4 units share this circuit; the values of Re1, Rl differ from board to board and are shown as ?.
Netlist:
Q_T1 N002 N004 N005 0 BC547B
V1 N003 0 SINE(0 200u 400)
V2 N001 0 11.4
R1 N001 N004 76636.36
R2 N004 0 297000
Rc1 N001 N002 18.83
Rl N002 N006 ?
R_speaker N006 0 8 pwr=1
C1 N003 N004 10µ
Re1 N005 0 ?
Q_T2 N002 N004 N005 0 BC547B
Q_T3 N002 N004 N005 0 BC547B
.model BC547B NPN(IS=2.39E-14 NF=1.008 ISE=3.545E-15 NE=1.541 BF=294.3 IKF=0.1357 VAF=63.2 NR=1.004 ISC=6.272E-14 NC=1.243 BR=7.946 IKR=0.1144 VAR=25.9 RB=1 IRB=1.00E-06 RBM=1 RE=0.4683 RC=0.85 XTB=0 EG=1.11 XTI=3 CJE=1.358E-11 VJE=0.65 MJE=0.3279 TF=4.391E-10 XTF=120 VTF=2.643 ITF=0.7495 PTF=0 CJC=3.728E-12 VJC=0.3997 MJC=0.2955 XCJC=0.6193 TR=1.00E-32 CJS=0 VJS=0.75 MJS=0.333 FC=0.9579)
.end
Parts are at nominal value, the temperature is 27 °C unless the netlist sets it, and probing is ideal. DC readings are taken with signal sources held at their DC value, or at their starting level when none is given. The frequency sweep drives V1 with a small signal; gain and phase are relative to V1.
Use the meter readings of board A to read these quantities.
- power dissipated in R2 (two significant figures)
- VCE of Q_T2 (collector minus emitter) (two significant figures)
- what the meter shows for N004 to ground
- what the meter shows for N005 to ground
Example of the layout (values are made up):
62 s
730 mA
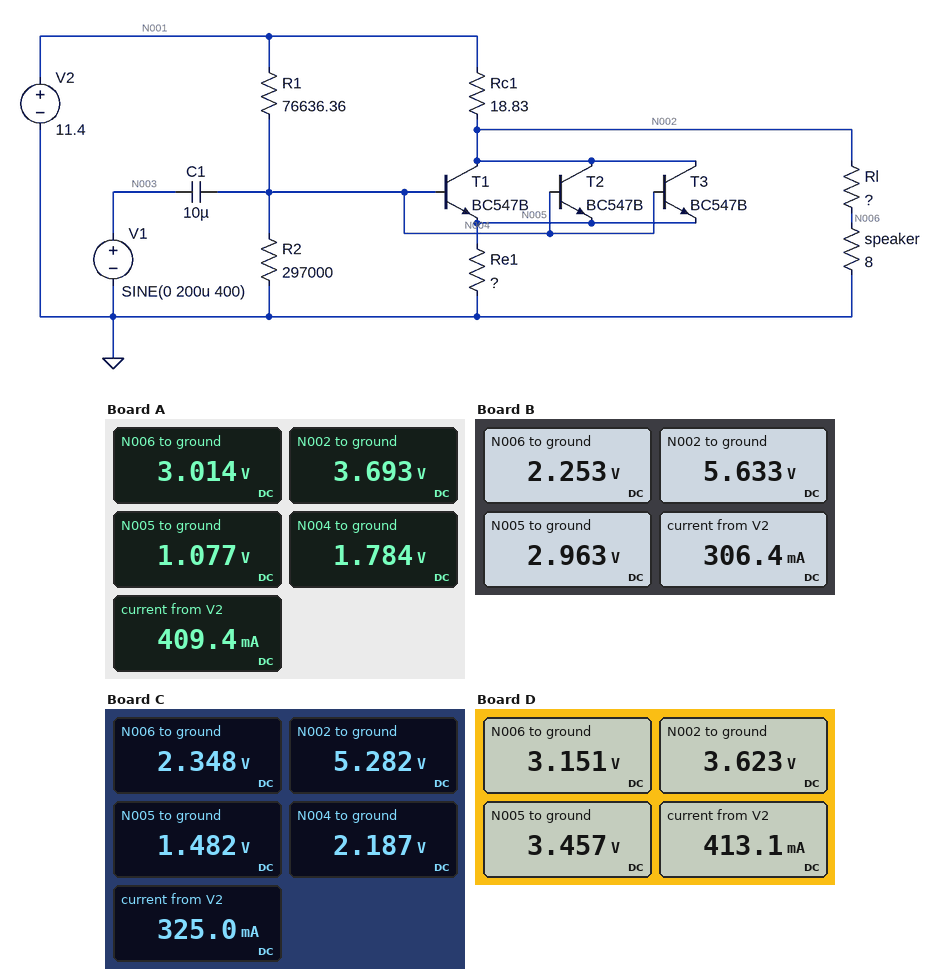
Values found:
11 µW
2.6 V
1.784 V
1.077 V
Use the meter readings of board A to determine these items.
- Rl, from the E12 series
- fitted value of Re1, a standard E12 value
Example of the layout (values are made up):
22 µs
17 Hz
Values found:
1.8 Ω
33 Ω
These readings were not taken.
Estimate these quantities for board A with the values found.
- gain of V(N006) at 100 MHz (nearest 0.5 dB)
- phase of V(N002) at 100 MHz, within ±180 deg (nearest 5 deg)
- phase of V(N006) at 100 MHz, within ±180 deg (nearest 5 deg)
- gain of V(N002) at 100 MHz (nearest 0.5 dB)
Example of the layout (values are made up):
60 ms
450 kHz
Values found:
-16.5 dB
150 deg
150 deg
-14.5 dB
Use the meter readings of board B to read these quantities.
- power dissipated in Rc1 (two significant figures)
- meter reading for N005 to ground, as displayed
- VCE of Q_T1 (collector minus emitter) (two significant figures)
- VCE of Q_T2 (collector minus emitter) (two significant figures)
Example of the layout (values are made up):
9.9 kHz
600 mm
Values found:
1.8 W
2.963 V
2.7 V
2.7 V
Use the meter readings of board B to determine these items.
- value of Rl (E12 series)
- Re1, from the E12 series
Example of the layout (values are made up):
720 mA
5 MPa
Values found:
12 Ω
120 Ω
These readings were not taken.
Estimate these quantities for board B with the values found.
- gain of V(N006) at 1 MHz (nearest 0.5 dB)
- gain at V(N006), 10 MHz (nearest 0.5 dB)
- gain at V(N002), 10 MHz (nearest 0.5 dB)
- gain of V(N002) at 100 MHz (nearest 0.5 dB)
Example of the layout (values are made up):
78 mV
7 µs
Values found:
-30.0 dB
-30.0 dB
-22.0 dB
-20.5 dB
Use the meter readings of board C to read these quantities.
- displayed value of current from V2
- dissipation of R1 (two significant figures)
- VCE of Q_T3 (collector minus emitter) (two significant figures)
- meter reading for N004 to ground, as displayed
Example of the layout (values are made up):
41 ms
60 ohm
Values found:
325.0 mA
1.1 mW
3.8 V
2.187 V
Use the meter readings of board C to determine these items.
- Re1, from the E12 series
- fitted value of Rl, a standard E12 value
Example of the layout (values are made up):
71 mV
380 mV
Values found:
47 Ω
10 Ω
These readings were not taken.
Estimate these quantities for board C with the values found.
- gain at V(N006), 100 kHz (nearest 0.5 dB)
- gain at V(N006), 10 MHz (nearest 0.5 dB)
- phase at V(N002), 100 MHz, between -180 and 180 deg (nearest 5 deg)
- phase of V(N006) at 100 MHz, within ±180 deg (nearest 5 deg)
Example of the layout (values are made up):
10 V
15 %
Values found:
-21.5 dB
-21.5 dB
145 deg
145 deg
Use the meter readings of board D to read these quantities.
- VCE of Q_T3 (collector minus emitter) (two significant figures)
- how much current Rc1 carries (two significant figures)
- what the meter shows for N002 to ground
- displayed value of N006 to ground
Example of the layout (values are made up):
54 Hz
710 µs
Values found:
170 mV
410 mA
3.623 V
3.151 V
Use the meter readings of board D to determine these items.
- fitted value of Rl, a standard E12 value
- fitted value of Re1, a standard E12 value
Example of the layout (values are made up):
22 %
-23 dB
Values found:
1.2 Ω
180 Ω
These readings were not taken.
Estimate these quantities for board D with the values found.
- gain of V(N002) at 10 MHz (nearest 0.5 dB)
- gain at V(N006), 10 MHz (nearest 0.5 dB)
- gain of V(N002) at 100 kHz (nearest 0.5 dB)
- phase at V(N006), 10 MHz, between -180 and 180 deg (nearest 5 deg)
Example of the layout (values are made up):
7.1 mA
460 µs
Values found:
-25.5 dB
-27.0 dB
-30.0 dB
125 deg
